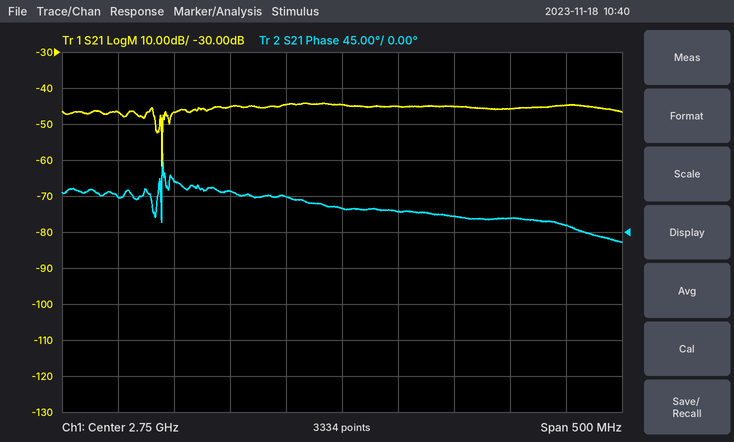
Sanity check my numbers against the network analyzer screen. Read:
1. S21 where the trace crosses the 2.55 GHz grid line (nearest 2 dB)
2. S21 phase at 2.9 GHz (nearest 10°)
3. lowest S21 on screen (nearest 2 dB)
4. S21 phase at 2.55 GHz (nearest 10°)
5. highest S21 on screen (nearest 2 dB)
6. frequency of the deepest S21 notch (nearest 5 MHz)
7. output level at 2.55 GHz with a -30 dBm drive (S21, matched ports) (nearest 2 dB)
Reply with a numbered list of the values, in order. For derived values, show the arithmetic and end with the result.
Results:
1. -46 dB
2. 20°
3. -62 dB
4. 40°
5. -44 dB
6. 2.590 GHz
7. -30 dBm + (-46 dB) = -76 dBm
